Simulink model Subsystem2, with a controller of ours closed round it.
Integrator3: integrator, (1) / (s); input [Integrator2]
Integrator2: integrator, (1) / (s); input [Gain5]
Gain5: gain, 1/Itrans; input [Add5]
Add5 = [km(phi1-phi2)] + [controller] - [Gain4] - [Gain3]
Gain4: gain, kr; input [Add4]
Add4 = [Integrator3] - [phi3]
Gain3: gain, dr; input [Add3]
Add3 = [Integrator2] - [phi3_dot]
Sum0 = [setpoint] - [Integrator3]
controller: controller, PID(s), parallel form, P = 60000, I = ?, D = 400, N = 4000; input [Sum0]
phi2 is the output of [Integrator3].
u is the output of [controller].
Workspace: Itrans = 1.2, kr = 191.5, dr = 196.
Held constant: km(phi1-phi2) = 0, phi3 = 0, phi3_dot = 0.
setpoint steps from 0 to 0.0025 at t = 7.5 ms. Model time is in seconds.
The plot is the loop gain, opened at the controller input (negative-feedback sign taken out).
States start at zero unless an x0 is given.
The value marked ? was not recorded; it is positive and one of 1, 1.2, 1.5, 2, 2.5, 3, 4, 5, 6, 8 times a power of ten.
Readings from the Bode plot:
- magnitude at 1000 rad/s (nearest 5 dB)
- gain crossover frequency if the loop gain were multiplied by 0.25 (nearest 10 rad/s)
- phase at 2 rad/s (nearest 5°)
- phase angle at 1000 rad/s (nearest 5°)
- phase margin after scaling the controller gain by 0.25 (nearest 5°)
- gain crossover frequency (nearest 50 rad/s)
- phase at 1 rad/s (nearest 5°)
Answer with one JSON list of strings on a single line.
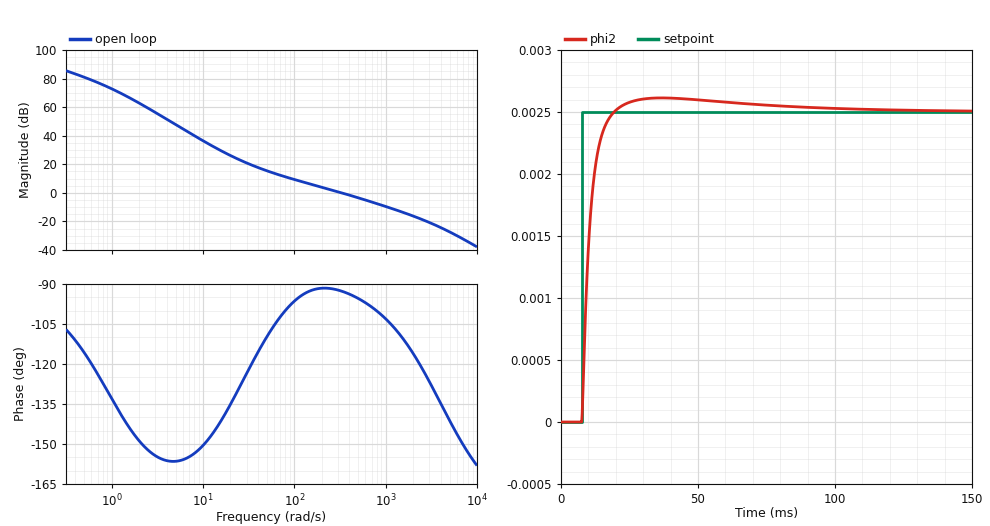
["-10 dB", "70 rad/s", "-150°", "-105°", "80°", "350 rad/s", "-135°"]
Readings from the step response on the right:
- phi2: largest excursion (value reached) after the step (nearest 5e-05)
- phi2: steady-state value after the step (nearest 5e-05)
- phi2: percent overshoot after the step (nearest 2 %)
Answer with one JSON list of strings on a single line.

["0.00260", "0.00250", "4 %"]
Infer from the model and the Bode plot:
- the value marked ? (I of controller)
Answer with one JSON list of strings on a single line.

["1.2e+06"]
